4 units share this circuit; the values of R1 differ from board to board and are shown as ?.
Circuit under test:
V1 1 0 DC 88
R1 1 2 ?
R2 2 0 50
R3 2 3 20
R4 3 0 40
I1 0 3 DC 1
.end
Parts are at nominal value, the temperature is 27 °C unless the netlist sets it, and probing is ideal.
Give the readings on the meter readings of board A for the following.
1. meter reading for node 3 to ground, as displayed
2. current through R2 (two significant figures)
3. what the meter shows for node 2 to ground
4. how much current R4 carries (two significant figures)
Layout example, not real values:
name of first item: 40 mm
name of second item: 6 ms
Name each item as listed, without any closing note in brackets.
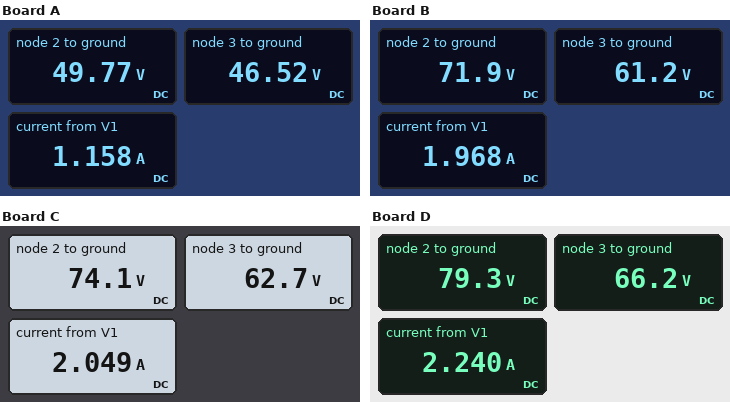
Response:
meter reading for node 3 to ground, as displayed: 46.52 V
current through R2: 1.0 A
what the meter shows for node 2 to ground: 49.77 V
how much current R4 carries: 1.2 A
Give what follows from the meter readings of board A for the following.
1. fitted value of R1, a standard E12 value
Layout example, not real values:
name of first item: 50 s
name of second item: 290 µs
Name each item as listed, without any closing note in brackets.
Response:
fitted value of R1, a standard E12 value: 33 Ω
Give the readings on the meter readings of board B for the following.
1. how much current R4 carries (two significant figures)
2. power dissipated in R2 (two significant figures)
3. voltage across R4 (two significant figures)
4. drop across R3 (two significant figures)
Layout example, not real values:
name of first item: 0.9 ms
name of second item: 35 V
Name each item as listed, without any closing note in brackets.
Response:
how much current R4 carries: 1.5 A
power dissipated in R2: 100 W
voltage across R4: 61 V
drop across R3: 11 V
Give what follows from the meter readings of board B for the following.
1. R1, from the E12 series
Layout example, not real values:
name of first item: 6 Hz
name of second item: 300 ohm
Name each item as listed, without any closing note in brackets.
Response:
R1, from the E12 series: 8.2 Ω
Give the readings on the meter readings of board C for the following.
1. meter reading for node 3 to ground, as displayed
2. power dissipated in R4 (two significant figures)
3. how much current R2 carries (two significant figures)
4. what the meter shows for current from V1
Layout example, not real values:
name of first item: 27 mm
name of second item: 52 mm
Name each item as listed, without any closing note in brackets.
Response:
meter reading for node 3 to ground, as displayed: 62.7 V
power dissipated in R4: 98 W
how much current R2 carries: 1.5 A
what the meter shows for current from V1: 2.049 A
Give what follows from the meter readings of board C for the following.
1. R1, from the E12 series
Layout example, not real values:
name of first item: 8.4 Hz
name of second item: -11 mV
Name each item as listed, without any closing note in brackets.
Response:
R1, from the E12 series: 6.8 Ω
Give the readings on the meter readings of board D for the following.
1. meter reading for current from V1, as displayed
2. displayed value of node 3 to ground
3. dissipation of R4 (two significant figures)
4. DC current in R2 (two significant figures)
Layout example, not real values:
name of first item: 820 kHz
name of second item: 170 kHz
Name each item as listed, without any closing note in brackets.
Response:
meter reading for current from V1, as displayed: 2.240 A
displayed value of node 3 to ground: 66.2 V
dissipation of R4: 110 W
DC current in R2: 1.6 A
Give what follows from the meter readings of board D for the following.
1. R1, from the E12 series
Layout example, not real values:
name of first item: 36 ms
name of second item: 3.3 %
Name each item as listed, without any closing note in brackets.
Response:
R1, from the E12 series: 3.9 Ω
